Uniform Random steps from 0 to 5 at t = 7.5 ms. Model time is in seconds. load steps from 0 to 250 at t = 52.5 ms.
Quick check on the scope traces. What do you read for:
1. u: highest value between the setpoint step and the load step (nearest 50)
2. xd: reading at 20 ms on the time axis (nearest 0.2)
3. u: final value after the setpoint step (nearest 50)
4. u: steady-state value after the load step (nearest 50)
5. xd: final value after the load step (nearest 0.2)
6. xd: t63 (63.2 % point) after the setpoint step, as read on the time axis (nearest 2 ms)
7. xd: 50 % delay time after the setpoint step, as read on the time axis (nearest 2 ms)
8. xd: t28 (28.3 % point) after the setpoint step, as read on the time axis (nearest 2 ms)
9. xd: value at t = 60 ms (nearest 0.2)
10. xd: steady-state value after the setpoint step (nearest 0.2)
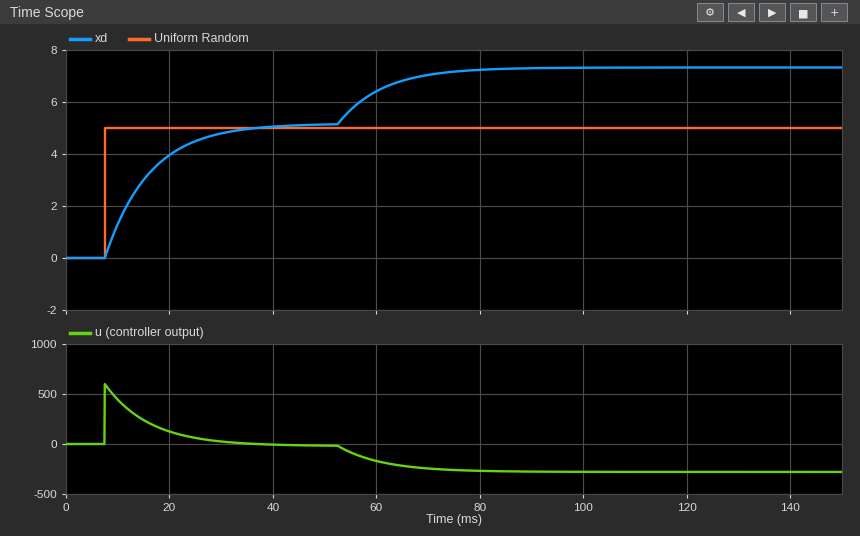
600
4.0
0
-300
7.4
16 ms
14 ms
10 ms
6.4
5.2
